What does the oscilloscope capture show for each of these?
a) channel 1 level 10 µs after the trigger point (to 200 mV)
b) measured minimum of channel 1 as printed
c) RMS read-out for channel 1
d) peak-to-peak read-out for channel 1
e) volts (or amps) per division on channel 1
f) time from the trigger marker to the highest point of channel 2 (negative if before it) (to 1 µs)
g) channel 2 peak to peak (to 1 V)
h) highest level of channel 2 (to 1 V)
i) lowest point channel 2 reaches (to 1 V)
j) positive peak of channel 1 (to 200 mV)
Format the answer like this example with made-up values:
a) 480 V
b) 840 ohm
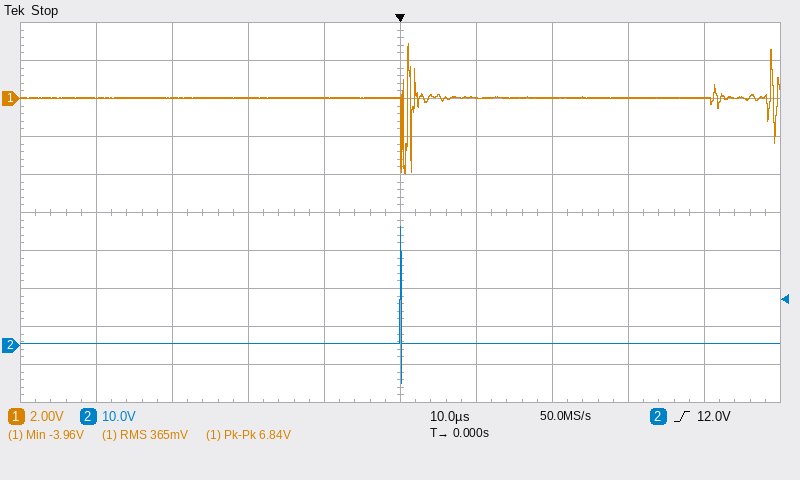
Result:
a) 0.0 V
b) -3.96 V
c) 365 mV
d) 6.84 V
e) 2 V
f) 0 µs
g) 41 V
h) 31 V
i) -10 V
j) 2.8 V
